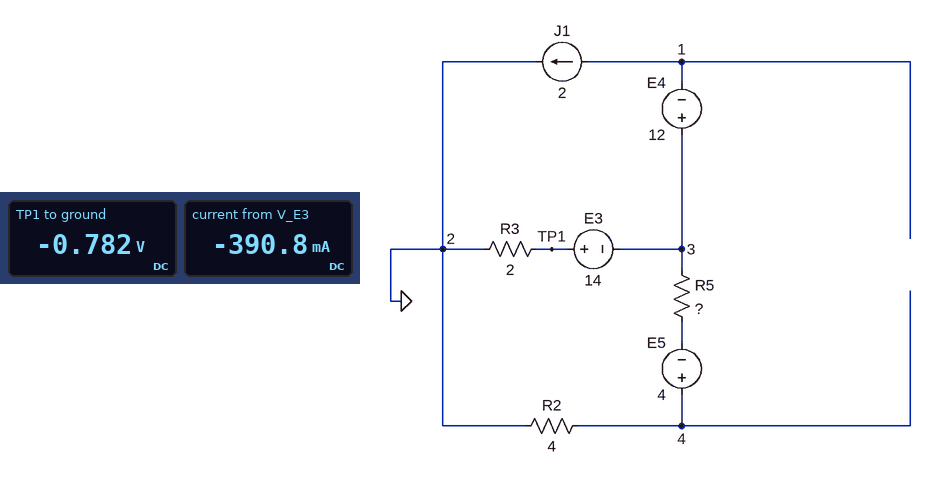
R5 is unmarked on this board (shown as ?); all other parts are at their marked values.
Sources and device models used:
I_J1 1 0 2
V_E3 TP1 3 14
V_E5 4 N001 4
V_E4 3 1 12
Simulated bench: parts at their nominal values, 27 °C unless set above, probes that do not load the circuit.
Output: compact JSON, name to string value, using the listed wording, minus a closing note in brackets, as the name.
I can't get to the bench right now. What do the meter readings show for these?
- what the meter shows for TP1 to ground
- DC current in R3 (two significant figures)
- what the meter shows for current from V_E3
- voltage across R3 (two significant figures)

{"what the meter shows for TP1 to ground": "-0.782 V", "DC current in R3": "390 mA", "what the meter shows for current from V_E3": "-390.8 mA", "voltage across R3": "780 mV"}
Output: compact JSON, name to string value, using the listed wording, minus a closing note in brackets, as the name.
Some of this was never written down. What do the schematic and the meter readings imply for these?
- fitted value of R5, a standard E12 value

{"fitted value of R5, a standard E12 value": "2.7 Ω"}
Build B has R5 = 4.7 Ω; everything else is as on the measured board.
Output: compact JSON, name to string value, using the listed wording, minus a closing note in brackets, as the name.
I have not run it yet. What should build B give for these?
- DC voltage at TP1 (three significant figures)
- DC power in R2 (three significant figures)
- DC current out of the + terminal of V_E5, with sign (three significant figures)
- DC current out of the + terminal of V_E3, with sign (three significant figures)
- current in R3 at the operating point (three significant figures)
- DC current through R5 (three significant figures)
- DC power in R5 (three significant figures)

{"DC voltage at TP1": "-1.38 V", "DC power in R2": "6.85 W", "DC current out of the + terminal of V_E5, with sign": "-1.31 A", "DC current out of the + terminal of V_E3, with sign": "-692 mA", "current in R3 at the operating point": "692 mA", "DC current through R5": "1.31 A", "DC power in R5": "8.05 W"}
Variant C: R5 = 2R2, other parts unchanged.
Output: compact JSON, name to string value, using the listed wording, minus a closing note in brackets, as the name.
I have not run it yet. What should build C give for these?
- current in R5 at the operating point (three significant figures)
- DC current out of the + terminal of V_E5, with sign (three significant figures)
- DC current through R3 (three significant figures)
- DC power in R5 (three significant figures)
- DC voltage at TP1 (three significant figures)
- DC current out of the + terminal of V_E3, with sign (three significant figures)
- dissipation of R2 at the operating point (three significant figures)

{"current in R5 at the operating point": "1.71 A", "DC current out of the + terminal of V_E5, with sign": "-1.71 A", "DC current through R3": "293 mA", "DC power in R5": "6.41 W", "DC voltage at TP1": "-585 mV", "DC current out of the + terminal of V_E3, with sign": "-293 mA", "dissipation of R2 at the operating point": "11.7 W"}
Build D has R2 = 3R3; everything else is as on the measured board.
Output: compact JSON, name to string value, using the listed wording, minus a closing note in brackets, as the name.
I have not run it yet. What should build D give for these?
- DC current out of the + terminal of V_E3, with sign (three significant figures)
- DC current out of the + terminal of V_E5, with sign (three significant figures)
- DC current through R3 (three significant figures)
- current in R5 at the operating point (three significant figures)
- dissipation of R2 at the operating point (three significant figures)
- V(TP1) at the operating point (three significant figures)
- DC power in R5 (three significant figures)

{"DC current out of the + terminal of V_E3, with sign": "-250 mA", "DC current out of the + terminal of V_E5, with sign": "-1.75 A", "DC current through R3": "250 mA", "current in R5 at the operating point": "1.75 A", "dissipation of R2 at the operating point": "10.1 W", "V(TP1) at the operating point": "-500 mV", "DC power in R5": "8.27 W"}
